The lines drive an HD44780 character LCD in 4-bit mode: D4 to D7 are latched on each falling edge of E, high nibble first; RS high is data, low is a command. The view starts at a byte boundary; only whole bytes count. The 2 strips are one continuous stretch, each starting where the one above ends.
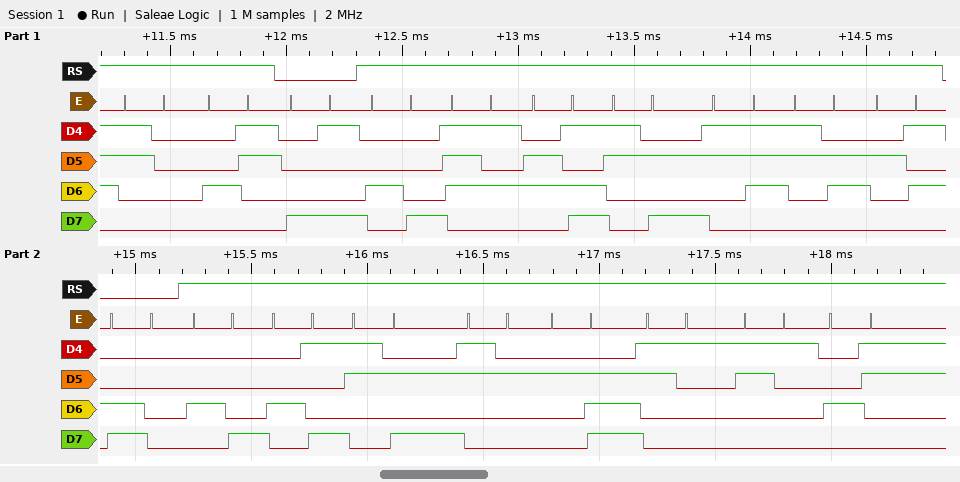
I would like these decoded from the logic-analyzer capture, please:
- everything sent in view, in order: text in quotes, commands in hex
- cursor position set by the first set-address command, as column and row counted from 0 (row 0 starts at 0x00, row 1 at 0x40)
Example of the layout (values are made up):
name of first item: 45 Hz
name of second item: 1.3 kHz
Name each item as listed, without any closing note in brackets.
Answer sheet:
everything sent in view, in order: text in quotes, commands in hex: "0C" 0x89 "Hum:76%" 0xC0 "HI:2.11C"
cursor position set by the first set-address command, as column and row counted from 0: column 9, row 0
